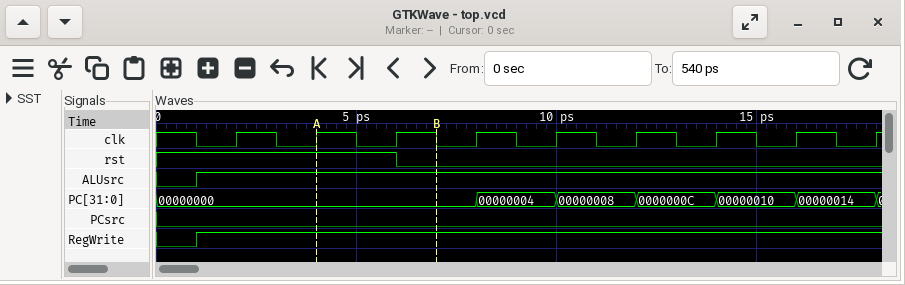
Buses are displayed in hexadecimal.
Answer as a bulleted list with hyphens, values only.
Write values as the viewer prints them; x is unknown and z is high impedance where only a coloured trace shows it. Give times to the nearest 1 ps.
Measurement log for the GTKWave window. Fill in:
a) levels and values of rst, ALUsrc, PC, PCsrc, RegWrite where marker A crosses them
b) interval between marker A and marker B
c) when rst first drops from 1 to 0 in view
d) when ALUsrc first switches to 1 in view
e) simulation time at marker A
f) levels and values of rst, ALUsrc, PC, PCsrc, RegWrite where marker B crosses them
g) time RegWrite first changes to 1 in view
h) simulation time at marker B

- rst=1, ALUsrc=1, PC=00000000, PCsrc=0, RegWrite=1
- 3 ps
- 6 ps
- 1 ps
- 4 ps
- rst=0, ALUsrc=1, PC=00000000, PCsrc=0, RegWrite=1
- 1 ps
- 7 ps
